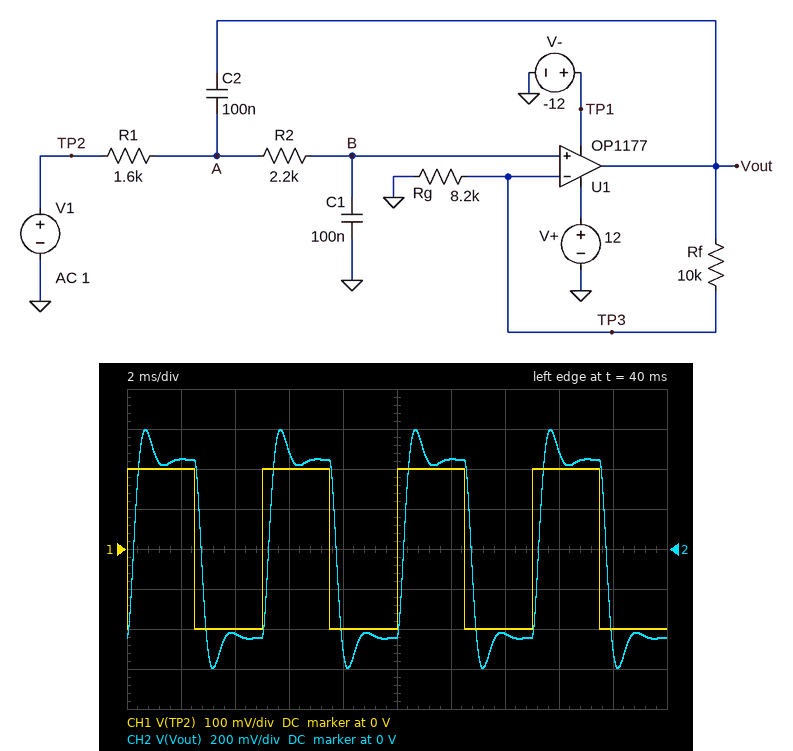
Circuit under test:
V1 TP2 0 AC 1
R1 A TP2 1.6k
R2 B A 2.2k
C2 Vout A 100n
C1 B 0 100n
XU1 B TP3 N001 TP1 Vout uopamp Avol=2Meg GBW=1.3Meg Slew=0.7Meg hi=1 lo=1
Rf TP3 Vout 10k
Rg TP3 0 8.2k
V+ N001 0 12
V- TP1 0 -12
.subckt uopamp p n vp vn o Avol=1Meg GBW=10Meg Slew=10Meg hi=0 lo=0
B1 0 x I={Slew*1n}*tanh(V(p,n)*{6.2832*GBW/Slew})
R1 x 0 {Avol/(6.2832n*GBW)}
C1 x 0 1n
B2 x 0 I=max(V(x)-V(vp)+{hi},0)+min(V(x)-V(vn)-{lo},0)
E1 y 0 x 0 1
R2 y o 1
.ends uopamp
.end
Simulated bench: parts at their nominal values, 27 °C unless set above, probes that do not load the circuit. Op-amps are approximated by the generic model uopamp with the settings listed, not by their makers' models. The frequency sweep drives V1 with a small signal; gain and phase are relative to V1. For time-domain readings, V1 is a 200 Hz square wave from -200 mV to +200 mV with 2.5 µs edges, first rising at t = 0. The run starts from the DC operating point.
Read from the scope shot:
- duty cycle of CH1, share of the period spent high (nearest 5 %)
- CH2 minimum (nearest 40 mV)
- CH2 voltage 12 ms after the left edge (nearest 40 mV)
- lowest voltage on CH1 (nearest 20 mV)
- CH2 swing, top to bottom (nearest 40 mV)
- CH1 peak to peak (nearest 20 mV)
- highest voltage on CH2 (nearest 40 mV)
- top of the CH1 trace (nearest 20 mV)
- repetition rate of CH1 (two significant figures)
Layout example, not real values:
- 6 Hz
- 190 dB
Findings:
- 50 %
- -600 mV
- 440 mV
- -200 mV
- 1.20 V
- 400 mV
- 600 mV
- 200 mV
- 200 Hz
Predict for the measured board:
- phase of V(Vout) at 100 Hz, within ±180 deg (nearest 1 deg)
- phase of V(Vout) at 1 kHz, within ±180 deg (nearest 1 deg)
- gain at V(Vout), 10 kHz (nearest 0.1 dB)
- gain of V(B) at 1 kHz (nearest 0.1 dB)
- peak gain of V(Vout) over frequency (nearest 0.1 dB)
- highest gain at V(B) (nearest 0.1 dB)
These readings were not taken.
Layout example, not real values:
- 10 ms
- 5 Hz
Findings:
- -7 deg
- -109 deg
- -35.9 dB
- -1.8 dB
- 8.3 dB
- 1.3 dB
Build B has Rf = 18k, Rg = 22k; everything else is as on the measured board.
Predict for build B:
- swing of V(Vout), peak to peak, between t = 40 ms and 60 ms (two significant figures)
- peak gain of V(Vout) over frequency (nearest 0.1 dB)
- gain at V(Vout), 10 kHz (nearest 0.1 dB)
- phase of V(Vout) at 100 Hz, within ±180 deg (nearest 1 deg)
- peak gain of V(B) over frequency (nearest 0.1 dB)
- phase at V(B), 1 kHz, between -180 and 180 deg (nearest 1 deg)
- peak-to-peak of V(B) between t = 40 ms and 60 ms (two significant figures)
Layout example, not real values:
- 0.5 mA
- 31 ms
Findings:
- 820 mV
- 5.3 dB
- -37.7 dB
- -9 deg
- 0.1 dB
- -104 deg
- 450 mV
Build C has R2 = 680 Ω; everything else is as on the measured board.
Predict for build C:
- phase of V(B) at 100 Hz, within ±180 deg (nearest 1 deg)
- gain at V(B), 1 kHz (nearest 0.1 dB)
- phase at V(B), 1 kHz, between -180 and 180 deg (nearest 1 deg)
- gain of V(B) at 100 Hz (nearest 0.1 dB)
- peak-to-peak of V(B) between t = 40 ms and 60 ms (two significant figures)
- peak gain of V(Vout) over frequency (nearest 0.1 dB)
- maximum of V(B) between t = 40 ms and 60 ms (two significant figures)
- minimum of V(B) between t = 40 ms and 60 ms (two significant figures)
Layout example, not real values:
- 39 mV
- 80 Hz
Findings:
- -1 deg
- 4.4 dB
- -20 deg
- 0 dB
- 890 mV
- 17.1 dB
- 440 mV
- -440 mV
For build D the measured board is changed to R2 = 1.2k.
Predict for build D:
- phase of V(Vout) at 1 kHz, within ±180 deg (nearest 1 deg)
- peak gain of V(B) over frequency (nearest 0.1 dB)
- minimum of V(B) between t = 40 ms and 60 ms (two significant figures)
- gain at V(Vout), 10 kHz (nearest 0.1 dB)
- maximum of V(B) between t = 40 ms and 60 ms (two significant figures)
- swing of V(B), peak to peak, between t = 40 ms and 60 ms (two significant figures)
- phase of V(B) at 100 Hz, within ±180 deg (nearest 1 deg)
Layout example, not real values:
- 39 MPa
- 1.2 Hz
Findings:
- -66 deg
- 4.7 dB
- -350 mV
- -30.6 dB
- 350 mV
- 690 mV
- -3 deg
